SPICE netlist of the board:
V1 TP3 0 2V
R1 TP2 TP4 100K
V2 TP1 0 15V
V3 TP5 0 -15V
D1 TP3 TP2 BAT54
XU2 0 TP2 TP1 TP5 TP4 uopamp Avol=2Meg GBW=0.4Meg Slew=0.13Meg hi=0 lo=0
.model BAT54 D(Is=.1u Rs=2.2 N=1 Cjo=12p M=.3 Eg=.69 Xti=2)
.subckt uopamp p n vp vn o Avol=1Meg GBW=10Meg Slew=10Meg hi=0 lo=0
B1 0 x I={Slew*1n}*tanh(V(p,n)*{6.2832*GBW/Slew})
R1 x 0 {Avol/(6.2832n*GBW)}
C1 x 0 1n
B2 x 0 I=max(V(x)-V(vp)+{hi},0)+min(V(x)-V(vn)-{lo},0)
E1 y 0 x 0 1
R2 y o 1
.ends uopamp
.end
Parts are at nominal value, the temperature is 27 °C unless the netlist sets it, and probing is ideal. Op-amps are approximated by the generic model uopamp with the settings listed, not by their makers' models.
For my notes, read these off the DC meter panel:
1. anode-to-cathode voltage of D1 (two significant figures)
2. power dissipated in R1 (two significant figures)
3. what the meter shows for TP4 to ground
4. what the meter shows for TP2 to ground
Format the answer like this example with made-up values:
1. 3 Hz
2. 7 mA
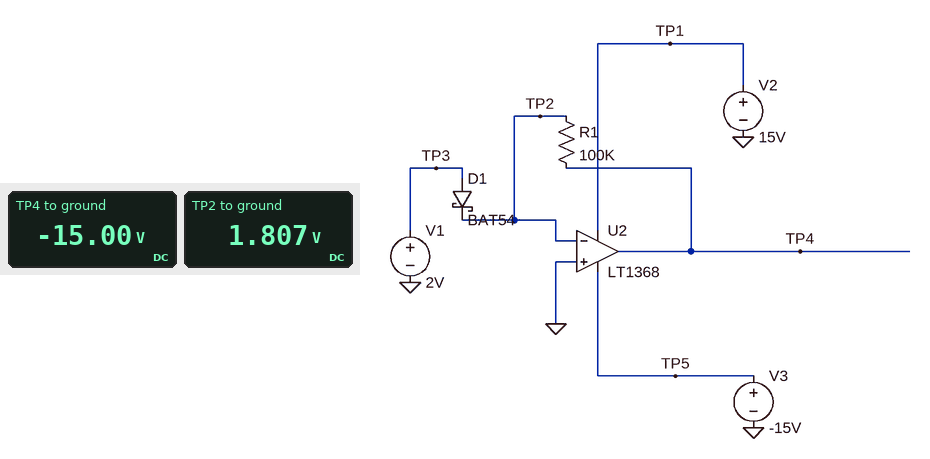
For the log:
1. 190 mV
2. 2.8 mW
3. -15.00 V
4. 1.807 V
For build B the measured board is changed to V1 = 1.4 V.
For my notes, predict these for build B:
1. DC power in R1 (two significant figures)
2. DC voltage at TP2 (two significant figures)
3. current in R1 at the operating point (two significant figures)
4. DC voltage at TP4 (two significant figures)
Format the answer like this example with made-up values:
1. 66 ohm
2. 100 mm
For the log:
1. 2.6 mW
2. 1.2 V
3. 160 µA
4. -15 V
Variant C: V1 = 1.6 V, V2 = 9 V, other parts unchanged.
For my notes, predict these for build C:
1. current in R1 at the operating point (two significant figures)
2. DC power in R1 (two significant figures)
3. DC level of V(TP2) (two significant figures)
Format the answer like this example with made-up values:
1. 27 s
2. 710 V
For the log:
1. 160 µA
2. 2.7 mW
3. 1.4 V
